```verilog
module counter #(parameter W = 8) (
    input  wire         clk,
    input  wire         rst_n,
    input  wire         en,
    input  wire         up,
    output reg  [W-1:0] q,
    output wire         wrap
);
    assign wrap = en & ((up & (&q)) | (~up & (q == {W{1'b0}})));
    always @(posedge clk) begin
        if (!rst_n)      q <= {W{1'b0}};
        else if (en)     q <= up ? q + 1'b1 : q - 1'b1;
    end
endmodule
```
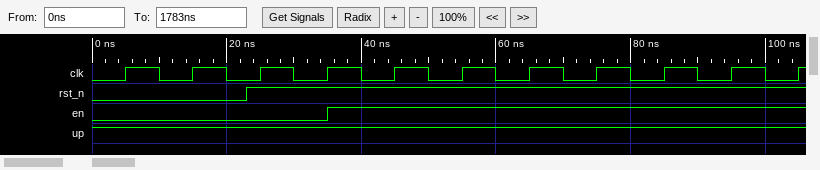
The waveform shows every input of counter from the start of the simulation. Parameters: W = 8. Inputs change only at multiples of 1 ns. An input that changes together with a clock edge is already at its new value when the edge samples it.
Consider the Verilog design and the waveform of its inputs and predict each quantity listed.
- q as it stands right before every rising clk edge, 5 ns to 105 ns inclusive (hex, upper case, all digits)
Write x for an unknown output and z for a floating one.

x, 00, 00, 00, 01, 02, 03, 04, 05, 06, 07
